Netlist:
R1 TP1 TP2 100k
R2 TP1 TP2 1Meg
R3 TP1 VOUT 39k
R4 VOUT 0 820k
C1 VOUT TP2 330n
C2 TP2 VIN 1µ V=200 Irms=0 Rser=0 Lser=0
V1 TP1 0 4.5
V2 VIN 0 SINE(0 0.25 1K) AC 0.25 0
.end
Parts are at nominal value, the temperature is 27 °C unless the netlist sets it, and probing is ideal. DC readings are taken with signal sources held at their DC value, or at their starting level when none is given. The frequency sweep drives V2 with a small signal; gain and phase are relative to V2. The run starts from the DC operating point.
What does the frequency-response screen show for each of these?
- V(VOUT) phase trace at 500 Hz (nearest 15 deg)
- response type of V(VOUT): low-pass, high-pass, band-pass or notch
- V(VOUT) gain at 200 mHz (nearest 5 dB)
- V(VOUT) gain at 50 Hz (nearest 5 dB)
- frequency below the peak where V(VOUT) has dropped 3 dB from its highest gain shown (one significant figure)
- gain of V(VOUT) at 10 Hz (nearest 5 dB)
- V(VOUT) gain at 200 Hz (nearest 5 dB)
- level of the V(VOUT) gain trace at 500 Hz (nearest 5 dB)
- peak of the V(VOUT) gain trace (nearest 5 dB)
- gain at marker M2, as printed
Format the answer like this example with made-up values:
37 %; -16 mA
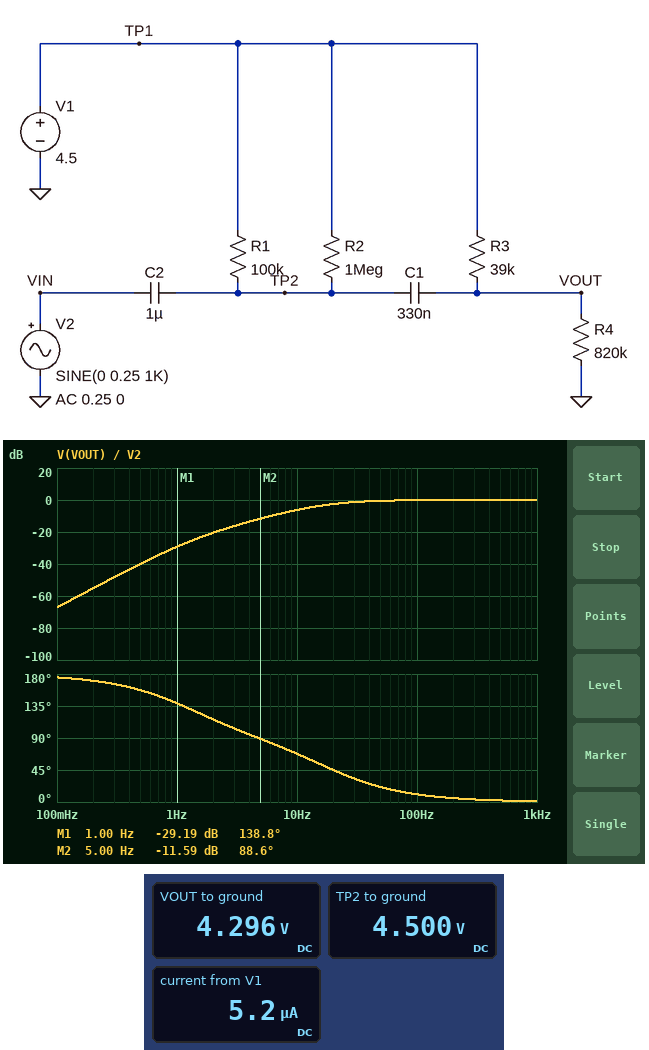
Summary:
0 deg; high-pass; -55 dB; 0 dB; 20 Hz; -5 dB; 0 dB; 0 dB; 0 dB; -11.59 dB
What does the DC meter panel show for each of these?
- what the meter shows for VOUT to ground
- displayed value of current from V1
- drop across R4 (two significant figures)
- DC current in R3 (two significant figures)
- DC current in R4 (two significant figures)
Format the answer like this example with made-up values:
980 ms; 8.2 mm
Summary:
4.296 V; 5.2 µA; 4.3 V; 5.2 µA; 5.2 µA
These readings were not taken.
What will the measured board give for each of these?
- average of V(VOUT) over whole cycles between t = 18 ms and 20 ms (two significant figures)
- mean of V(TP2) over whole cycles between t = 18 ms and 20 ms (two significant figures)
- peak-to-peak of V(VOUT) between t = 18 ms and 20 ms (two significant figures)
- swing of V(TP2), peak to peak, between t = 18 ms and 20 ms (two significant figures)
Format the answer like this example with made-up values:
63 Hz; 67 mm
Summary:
4.3 V; 4.5 V; 500 mV; 500 mV
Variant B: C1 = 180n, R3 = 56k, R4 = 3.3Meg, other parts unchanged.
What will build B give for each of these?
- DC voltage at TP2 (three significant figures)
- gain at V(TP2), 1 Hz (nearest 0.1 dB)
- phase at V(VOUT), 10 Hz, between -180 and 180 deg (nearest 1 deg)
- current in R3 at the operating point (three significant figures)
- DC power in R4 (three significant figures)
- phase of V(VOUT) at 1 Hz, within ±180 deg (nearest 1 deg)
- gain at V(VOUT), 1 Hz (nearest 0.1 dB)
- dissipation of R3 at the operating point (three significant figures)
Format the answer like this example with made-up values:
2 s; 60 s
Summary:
4.50 V; -6.5 dB; 71 deg; 1.34 µA; 5.93 µW; 143 deg; -30.7 dB; 101 nW
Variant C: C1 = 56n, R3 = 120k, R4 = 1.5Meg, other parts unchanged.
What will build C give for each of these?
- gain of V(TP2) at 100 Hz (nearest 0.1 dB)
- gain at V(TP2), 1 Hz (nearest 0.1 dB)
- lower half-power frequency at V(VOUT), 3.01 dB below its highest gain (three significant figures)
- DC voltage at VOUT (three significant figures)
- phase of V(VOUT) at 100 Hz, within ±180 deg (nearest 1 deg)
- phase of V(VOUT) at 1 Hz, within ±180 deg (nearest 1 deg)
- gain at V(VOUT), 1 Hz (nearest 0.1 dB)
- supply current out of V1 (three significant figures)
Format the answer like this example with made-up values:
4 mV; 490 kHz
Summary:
0 dB; -6.2 dB; 27.2 Hz; 4.17 V; 16 deg; 147 deg; -34.4 dB; 2.78 µA
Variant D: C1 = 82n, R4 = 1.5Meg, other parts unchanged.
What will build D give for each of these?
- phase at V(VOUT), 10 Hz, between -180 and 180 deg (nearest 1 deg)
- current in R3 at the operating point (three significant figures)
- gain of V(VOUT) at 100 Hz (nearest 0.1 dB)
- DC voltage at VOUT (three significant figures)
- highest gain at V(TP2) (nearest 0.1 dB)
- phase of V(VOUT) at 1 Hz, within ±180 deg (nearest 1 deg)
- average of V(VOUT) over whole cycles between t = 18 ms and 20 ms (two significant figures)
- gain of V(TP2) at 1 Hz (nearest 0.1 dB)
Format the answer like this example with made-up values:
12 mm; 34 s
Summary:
89 deg; 2.92 µA; -1.2 dB; 4.39 V; 0 dB; 147 deg; 4.4 V; -6.3 dB
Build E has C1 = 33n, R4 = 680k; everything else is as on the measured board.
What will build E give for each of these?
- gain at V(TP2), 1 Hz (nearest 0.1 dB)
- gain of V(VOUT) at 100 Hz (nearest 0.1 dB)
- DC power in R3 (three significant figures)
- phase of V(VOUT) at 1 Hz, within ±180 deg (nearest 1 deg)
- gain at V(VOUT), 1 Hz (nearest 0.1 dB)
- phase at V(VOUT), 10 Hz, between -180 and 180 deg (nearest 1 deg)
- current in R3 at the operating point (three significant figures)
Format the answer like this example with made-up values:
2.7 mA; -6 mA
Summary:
-6.2 dB; -4.5 dB; 1.53 µW; 149 deg; -48.5 dB; 95 deg; 6.26 µA
